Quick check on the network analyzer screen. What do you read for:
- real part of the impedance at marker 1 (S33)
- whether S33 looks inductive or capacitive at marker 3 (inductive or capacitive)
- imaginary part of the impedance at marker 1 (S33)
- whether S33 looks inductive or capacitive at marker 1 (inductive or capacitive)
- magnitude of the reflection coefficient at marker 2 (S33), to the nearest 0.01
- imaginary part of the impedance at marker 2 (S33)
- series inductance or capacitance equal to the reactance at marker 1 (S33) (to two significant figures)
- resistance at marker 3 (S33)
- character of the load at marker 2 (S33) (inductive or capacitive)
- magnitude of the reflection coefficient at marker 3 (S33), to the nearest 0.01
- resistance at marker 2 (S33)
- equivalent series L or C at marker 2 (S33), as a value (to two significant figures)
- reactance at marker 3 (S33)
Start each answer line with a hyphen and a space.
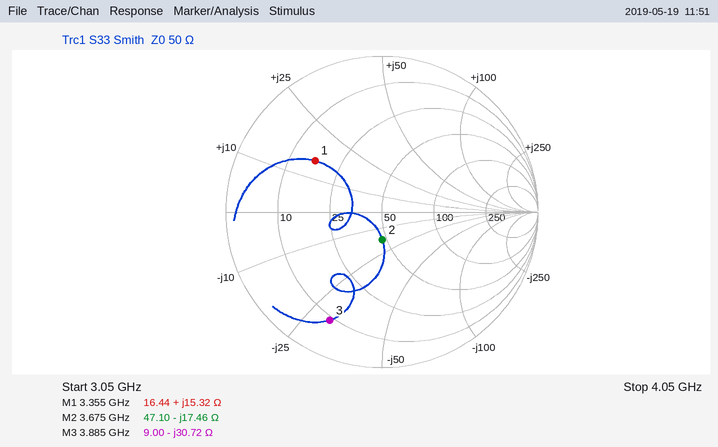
- 16.44 Ω
- capacitive
- +15.32 Ω
- inductive
- 0.18
- -17.46 Ω
- 730 pH
- 9.00 Ω
- capacitive
- 0.77
- 47.10 Ω
- 2.5 pF
- -30.72 Ω
